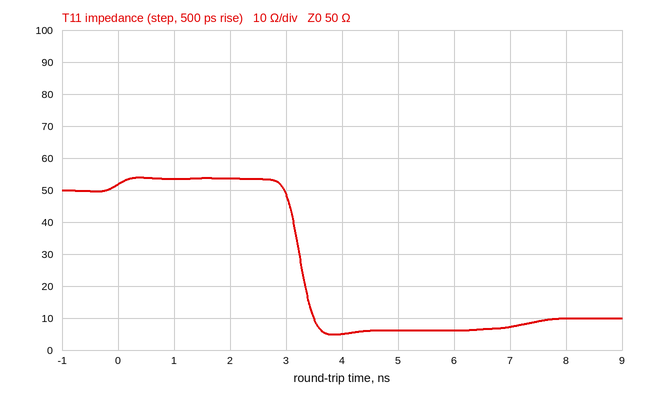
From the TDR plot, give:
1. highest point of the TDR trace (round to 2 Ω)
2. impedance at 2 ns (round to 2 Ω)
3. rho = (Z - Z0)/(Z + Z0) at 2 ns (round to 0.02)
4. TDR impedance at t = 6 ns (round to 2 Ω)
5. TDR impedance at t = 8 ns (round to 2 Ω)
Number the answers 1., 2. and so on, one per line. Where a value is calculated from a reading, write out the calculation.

1. 54 Ω
2. 54 Ω
3. (54 − 50)/(54 + 50) ≈ +0.04
4. 6 Ω
5. 10 Ω
